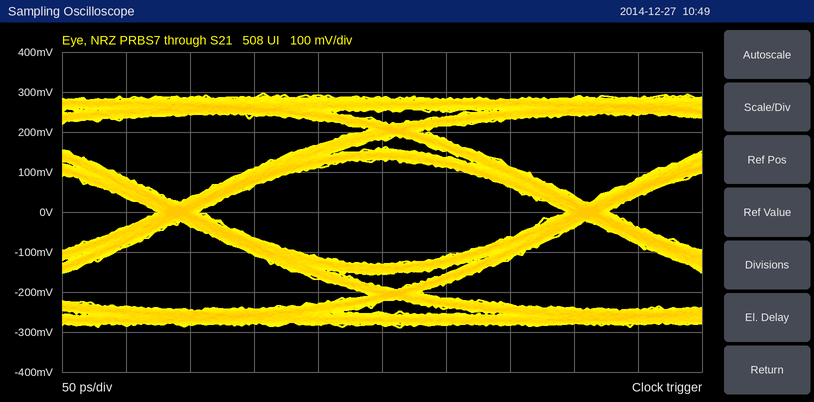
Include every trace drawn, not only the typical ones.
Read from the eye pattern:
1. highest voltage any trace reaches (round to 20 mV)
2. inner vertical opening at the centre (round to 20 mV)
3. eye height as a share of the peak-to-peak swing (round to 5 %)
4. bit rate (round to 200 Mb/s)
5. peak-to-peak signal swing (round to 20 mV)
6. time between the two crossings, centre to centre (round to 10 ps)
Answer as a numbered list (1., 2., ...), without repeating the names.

1. 300 mV
2. 260 mV
3. 45 %
4. 3.2 Gb/s
5. 580 mV
6. 320 ps
